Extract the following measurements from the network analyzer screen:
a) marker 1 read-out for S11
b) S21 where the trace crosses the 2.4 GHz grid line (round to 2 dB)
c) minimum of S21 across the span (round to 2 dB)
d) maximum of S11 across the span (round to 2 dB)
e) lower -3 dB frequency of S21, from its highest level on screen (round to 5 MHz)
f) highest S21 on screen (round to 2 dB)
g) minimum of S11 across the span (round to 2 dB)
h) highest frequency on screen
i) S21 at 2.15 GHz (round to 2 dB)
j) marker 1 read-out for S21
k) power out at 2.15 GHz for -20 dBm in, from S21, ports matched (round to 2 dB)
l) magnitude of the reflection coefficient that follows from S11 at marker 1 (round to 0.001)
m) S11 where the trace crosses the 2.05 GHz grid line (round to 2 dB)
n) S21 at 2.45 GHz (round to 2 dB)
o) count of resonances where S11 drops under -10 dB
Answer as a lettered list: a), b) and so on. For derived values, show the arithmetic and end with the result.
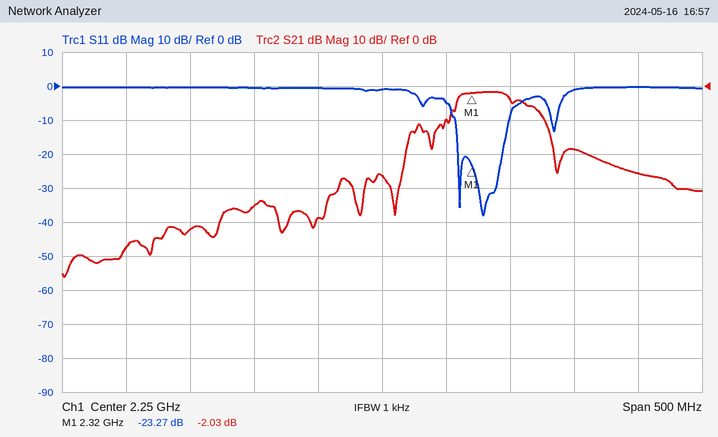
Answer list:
a) -23.27 dB
b) -18 dB
c) -56 dB
d) 0 dB
e) 2.310 GHz
f) -2 dB
g) -38 dB
h) 2.5 GHz
i) -36 dB
j) -2.03 dB
k) -20 dBm + (-36 dB) = -56 dBm
l) 10^(-23.27/20) ≈ 0.069
m) 0 dB
n) -26 dB
o) 3
